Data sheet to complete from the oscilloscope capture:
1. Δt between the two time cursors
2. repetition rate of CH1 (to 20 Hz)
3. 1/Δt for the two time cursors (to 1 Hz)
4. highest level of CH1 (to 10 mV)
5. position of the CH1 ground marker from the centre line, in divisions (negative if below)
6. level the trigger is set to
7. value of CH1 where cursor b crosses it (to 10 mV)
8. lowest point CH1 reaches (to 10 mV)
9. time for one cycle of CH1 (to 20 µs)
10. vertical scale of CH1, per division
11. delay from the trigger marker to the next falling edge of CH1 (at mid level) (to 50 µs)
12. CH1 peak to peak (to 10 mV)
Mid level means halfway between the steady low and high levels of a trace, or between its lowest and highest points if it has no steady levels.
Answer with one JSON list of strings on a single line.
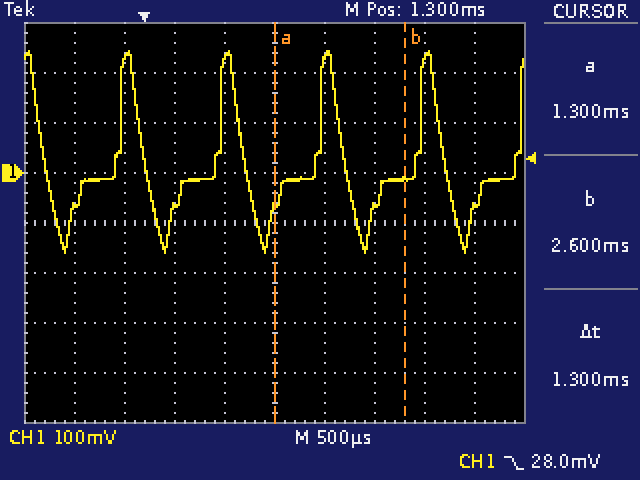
["1.3 ms", "1.00 kHz", "769 Hz", "240 mV", "+1.0 div", "28.0 mV", "-10 mV", "-160 mV", "1.00 ms", "100 mV", "1.00 ms", "400 mV"]
